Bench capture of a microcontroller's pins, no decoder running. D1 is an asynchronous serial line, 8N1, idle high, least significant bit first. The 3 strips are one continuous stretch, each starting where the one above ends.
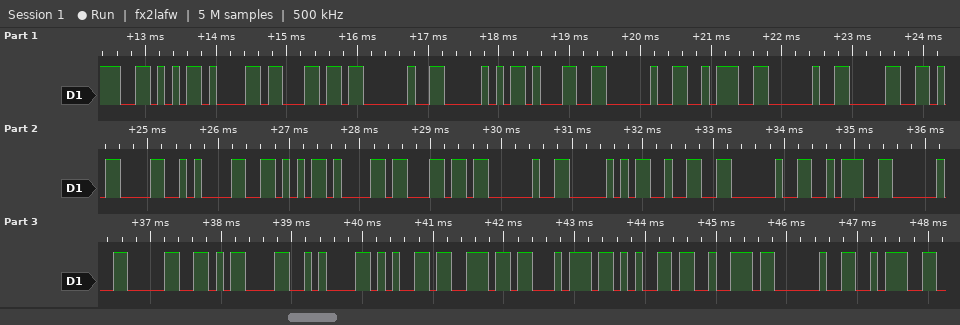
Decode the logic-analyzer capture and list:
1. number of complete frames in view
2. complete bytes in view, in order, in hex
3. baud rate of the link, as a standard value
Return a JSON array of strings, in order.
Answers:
["31", "0x56 0x61 0x6C 0x20 0x50 0x31 0x20 0x3A 0x20 0x30 0x0D 0x0A 0x56 0x61 0x6C 0x20 0x50 0x32 0x20 0x3A 0x20 0x30 0x0D 0x0A 0x65 0x6E 0x74 0x65 0x72 0x20 0x3A", "9600 baud"]
